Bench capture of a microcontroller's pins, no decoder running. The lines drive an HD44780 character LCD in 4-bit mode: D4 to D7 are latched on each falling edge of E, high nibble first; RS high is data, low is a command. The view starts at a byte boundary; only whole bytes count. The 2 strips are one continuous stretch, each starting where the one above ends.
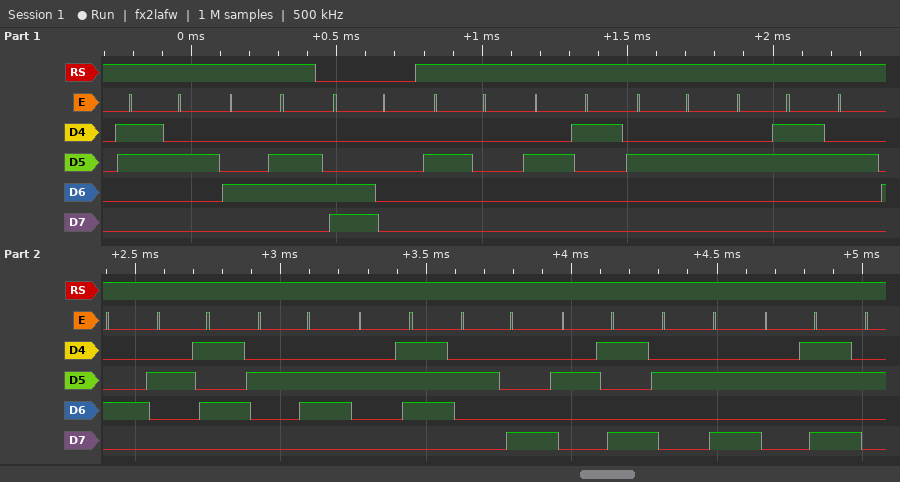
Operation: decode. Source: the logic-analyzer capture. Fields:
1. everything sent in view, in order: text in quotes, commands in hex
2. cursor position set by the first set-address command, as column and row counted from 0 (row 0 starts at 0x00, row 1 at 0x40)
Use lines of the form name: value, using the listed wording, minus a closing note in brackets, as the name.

everything sent in view, in order: text in quotes, commands in hex: "2F" 0xC0 " !\"#$%&'()*+"
cursor position set by the first set-address command, as column and row counted from 0: column 0, row 1
